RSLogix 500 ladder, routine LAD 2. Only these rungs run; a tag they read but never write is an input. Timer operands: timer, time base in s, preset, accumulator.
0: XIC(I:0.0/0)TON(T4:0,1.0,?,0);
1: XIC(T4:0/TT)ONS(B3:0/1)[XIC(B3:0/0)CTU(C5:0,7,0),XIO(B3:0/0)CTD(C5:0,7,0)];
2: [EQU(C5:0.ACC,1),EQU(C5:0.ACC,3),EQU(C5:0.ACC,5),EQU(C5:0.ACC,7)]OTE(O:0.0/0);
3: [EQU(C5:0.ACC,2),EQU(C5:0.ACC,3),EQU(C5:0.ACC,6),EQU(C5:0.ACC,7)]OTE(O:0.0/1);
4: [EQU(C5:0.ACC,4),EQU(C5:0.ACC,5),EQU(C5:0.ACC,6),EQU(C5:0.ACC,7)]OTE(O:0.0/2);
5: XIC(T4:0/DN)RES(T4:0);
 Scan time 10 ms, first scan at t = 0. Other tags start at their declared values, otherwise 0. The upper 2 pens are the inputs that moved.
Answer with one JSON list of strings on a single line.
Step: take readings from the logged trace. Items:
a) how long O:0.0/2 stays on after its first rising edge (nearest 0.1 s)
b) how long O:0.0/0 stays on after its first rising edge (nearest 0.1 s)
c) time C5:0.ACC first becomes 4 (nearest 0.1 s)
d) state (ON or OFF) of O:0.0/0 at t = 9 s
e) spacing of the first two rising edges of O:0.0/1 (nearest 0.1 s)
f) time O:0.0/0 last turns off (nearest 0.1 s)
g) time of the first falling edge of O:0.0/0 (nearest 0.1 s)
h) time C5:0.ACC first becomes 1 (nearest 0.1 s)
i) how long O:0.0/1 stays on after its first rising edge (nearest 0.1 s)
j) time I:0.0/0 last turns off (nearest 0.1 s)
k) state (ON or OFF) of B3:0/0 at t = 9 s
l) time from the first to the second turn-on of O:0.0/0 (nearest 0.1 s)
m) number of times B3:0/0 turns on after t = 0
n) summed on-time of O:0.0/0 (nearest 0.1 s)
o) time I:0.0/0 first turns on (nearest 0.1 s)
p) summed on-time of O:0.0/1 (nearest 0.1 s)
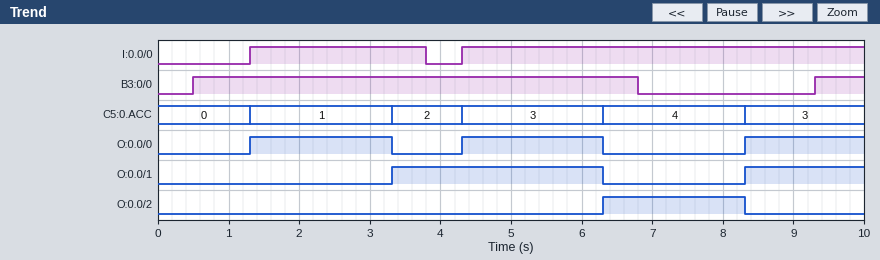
["2.0 s", "2.0 s", "6.3 s", "ON", "5.0 s", "6.3 s", "3.3 s", "1.3 s", "3.0 s", "3.8 s", "OFF", "3.0 s", "2", "5.7 s", "1.3 s", "4.7 s"]
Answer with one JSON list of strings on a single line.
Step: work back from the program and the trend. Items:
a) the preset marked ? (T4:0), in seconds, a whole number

["2 s"]
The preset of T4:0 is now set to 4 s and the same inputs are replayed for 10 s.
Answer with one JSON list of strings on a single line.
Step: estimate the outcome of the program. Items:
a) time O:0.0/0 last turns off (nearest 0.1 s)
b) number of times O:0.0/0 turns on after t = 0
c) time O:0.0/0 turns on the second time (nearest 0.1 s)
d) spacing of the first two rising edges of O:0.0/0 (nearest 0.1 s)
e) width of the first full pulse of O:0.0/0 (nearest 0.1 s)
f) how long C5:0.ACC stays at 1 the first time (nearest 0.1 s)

["4.3 s", "2", "8.3 s", "7.0 s", "3.0 s", "3.0 s"]
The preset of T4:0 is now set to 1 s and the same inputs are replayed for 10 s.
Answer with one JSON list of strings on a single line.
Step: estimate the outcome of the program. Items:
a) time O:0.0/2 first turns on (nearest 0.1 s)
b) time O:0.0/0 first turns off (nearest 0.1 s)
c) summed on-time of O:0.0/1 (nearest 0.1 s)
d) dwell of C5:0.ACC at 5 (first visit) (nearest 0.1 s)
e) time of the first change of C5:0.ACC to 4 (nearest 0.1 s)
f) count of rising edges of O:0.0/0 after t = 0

["4.3 s", "2.3 s", "3.0 s", "1.0 s", "4.3 s", "5"]
